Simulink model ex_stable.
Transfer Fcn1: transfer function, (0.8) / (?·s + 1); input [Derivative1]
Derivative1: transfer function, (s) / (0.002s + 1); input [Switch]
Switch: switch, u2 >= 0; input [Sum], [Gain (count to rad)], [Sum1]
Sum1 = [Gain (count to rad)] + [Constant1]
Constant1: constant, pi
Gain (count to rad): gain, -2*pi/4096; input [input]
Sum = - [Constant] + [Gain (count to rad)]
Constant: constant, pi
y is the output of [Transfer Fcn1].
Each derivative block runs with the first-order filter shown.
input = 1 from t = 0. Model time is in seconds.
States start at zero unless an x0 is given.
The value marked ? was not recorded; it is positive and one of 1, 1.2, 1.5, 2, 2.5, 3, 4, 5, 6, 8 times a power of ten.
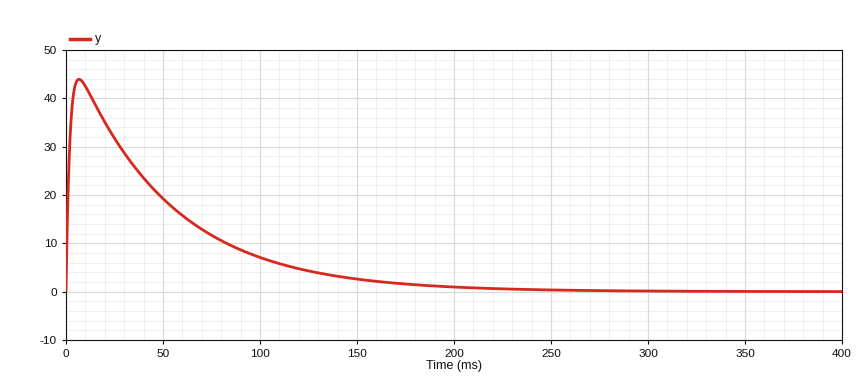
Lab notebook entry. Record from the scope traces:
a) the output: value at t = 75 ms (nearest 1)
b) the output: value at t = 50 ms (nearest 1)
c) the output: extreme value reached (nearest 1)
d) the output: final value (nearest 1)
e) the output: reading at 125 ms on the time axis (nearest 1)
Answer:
12
19
44
0
4
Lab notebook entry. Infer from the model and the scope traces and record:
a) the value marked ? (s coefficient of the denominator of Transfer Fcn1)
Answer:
0.05
